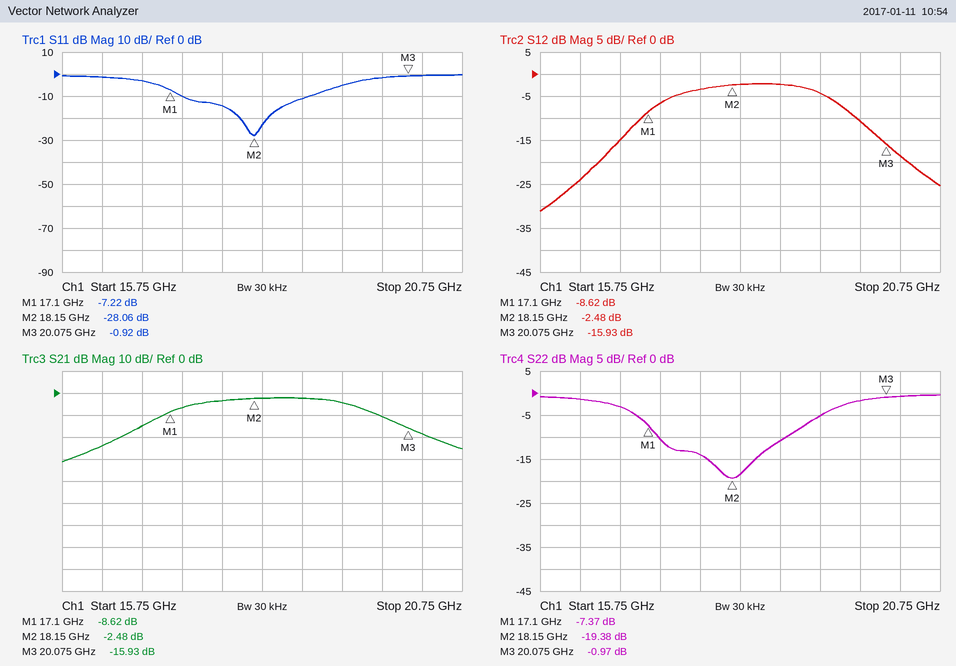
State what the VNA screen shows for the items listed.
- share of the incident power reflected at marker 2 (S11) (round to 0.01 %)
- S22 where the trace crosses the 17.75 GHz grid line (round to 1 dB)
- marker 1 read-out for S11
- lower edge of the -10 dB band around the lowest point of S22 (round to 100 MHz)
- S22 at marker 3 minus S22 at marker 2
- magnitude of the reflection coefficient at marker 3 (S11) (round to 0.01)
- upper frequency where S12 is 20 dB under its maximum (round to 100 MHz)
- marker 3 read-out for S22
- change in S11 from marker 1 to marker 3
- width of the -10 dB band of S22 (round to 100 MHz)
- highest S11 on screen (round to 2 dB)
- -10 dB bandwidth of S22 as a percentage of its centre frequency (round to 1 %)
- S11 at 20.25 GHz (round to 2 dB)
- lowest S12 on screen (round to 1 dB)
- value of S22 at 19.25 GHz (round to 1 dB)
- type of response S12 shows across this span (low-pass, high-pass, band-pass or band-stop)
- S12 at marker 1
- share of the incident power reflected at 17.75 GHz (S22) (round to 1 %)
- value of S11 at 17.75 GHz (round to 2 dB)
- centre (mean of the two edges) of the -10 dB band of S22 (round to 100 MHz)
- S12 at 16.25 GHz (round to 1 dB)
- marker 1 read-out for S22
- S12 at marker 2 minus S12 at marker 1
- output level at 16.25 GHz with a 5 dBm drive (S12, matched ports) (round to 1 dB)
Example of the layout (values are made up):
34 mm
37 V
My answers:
0.16 %
-14 dB
-7.22 dB
17.2 GHz
18.41 dB
0.90
20.5 GHz
-0.97 dB
6.30 dB
1.6 GHz
0 dB
9 %
0 dB
-31 dB
-5 dB
band-pass
-8.62 dB
4 %
-14 dB
18.0 GHz
-24 dB
-7.37 dB
6.14 dB
-19 dBm
